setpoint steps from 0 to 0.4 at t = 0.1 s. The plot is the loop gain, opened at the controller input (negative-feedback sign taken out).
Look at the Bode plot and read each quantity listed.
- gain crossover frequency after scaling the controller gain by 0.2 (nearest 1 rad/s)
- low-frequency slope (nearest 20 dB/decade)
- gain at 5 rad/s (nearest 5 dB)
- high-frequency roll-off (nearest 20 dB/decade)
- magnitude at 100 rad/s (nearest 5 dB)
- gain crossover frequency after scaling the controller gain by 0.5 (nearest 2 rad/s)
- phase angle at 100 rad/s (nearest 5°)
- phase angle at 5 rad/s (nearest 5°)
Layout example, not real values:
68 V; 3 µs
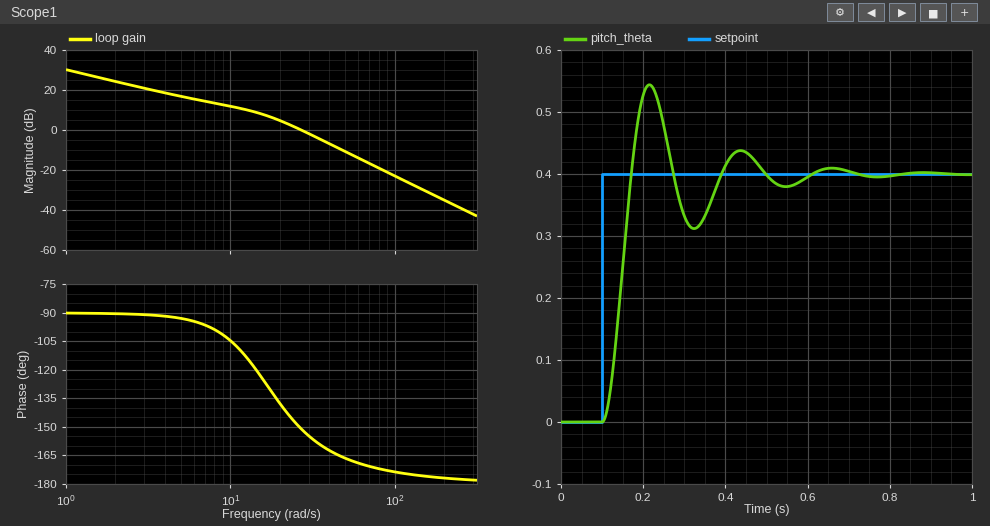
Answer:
7 rad/s; -20 dB/decade; 15 dB; -40 dB/decade; -25 dB; 18 rad/s; -175°; -95°
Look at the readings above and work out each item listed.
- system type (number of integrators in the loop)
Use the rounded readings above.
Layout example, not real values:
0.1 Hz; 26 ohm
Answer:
1
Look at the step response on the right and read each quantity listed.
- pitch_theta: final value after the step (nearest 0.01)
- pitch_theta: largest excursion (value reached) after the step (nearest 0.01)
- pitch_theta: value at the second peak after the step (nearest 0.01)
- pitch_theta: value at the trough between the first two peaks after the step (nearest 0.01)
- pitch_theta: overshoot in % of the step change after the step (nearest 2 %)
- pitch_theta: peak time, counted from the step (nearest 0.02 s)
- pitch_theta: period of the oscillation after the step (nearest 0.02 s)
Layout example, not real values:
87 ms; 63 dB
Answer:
0.40; 0.54; 0.44; 0.31; 36 %; 0.12 s; 0.22 s
